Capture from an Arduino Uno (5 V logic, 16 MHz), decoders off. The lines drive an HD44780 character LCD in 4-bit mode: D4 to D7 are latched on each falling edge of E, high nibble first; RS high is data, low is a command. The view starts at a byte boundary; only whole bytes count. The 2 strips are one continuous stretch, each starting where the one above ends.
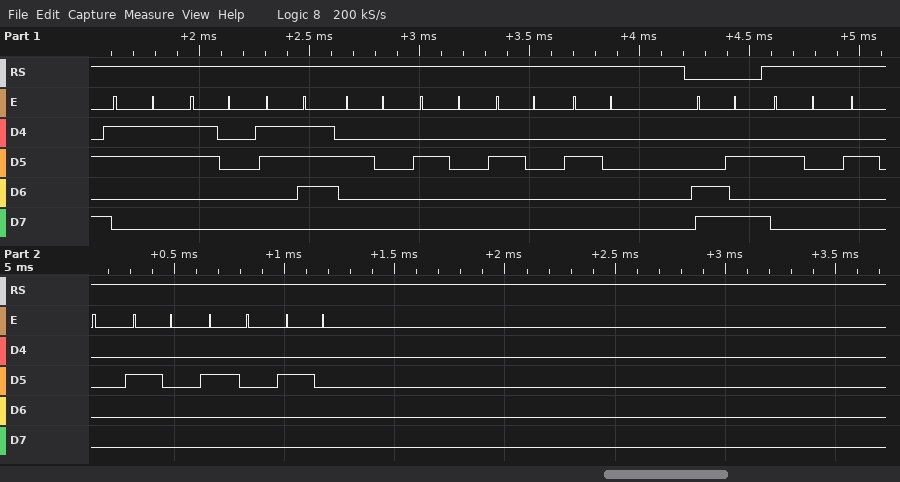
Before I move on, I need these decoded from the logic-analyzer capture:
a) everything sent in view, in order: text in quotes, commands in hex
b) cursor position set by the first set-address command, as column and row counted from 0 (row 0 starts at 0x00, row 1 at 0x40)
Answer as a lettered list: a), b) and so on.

a) "307    " 0xCA "     "
b) column 10, row 1
